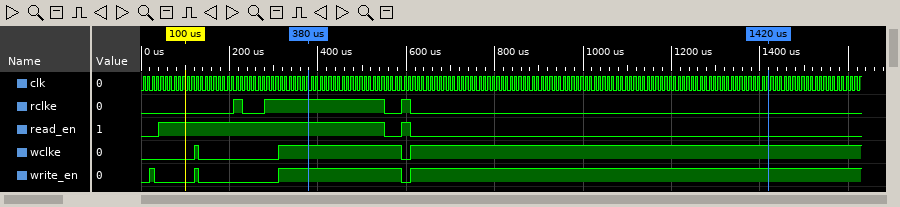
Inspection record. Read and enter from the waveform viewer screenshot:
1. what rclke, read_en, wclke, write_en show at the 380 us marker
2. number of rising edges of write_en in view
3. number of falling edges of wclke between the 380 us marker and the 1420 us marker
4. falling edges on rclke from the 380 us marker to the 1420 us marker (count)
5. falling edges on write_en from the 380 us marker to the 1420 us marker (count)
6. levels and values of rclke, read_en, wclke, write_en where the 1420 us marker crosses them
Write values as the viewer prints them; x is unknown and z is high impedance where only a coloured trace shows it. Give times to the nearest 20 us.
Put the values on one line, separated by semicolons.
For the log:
rclke=1, read_en=1, wclke=1, write_en=1; 4; 1; 2; 1; rclke=0, read_en=0, wclke=1, write_en=1
